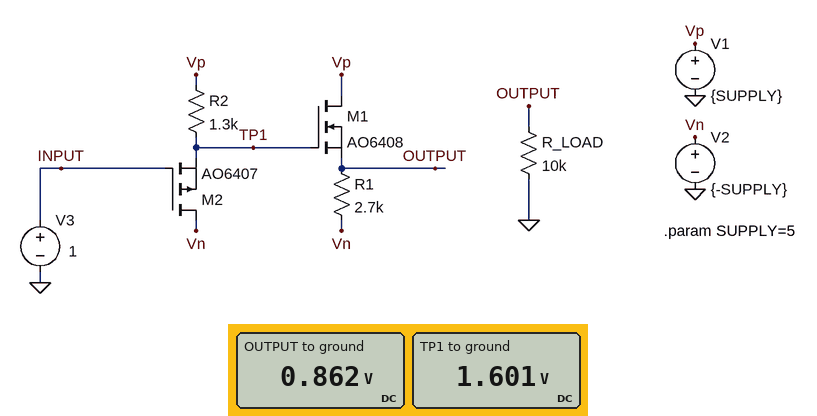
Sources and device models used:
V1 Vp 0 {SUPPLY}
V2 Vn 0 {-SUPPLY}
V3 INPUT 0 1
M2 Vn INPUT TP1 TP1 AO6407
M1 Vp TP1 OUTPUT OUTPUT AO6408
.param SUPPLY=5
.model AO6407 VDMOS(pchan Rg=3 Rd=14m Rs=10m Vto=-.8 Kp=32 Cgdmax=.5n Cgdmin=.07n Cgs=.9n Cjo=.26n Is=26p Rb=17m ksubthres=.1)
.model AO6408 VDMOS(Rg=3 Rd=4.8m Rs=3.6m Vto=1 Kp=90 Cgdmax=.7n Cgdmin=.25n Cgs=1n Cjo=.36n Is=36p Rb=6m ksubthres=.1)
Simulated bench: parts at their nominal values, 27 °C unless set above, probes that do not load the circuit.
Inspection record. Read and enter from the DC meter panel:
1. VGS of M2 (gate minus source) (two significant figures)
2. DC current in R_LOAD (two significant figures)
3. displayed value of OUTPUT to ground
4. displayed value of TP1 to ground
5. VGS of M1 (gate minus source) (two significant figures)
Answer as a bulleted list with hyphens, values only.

- -600 mV
- 86 µA
- 0.862 V
- 1.601 V
- 740 mV
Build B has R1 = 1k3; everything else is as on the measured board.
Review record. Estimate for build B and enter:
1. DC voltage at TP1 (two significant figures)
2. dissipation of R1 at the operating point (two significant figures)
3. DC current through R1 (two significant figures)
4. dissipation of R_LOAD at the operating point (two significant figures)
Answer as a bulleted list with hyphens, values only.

- 1.6 V
- 26 mW
- 4.5 mA
- 68 µW
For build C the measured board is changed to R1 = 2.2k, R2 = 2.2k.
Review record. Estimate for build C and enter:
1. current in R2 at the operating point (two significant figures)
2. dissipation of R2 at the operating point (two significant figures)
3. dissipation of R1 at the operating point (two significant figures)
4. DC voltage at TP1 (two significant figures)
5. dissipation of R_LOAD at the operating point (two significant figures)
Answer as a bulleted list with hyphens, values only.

- 1.6 mA
- 5.3 mW
- 15 mW
- 1.6 V
- 68 µW
